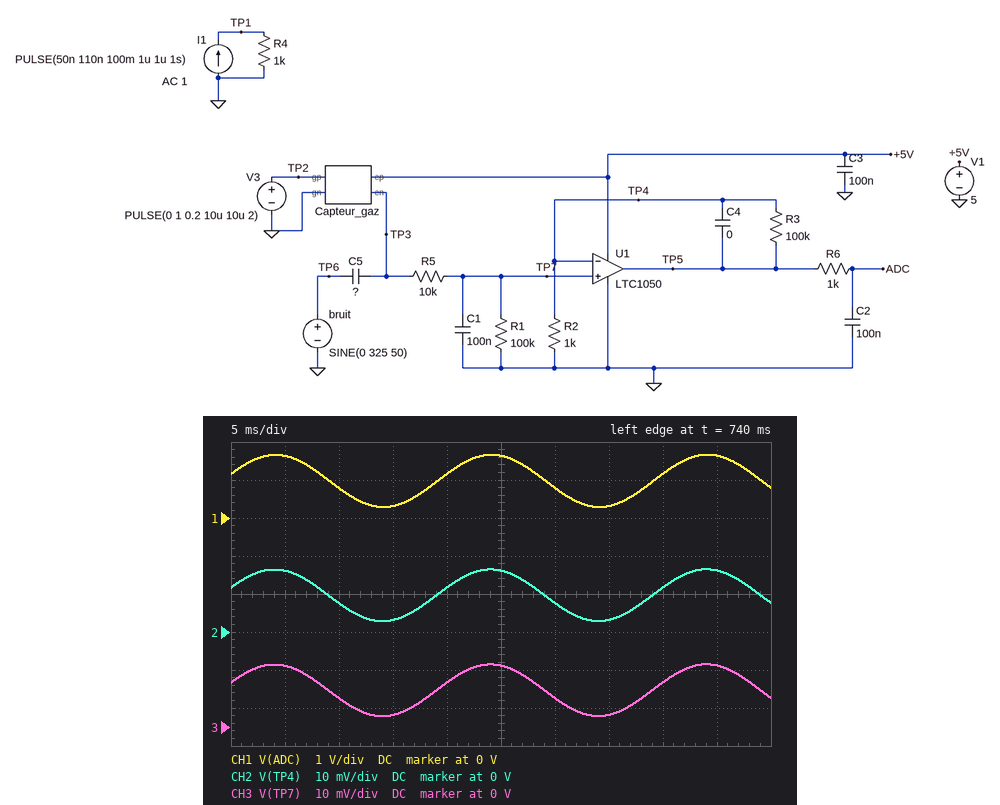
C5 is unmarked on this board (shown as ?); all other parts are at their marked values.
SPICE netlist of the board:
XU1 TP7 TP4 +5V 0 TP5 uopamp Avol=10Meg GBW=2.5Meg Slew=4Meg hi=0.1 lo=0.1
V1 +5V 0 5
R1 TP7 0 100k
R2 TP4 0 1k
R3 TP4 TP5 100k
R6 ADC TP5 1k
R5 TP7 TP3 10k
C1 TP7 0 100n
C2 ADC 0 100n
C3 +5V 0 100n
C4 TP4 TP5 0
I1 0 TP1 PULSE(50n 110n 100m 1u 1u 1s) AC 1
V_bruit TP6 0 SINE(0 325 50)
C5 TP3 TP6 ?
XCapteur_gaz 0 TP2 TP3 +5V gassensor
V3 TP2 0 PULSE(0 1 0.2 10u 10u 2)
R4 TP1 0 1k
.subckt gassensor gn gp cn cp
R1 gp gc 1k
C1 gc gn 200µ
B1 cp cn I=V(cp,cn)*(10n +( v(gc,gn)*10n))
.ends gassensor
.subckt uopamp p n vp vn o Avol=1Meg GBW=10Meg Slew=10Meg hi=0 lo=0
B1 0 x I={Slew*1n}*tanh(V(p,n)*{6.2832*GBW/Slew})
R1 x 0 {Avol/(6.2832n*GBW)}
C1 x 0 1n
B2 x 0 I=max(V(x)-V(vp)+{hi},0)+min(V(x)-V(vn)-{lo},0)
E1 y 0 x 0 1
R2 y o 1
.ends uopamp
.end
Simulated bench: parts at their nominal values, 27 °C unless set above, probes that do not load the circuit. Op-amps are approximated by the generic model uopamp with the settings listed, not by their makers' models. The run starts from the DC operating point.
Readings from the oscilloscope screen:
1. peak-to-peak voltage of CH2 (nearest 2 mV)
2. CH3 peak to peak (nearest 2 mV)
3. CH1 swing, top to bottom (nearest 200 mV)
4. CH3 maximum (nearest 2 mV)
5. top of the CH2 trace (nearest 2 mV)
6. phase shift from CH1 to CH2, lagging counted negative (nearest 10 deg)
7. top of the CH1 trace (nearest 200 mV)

14 mV
14 mV
1.4 V
16 mV
16 mV
0 deg
1.6 V
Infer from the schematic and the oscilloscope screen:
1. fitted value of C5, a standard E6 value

2.2 pF
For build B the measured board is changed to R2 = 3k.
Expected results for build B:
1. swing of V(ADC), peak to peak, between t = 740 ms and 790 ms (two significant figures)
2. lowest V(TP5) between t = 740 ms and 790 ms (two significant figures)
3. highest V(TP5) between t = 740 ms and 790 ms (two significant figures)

470 mV
100 mV
570 mV
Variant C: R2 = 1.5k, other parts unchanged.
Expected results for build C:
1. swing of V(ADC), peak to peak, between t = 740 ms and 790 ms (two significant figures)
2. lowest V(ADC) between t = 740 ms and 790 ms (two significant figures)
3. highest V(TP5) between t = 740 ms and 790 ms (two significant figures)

920 mV
190 mV
1.1 V
